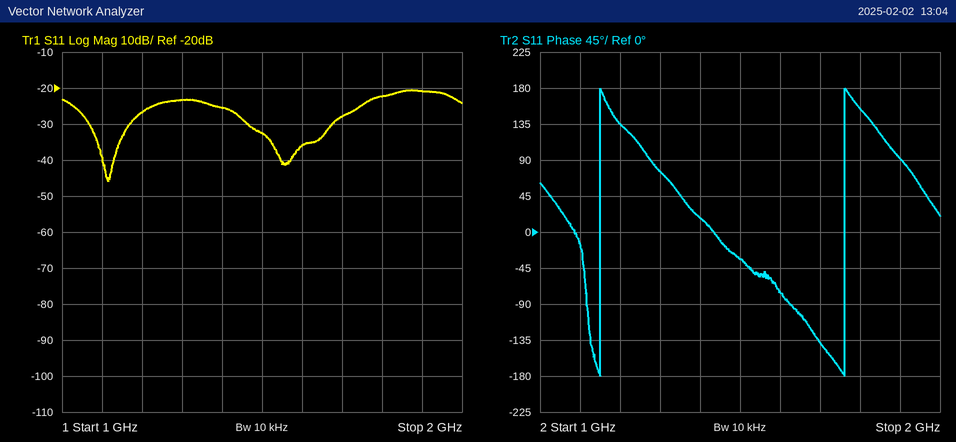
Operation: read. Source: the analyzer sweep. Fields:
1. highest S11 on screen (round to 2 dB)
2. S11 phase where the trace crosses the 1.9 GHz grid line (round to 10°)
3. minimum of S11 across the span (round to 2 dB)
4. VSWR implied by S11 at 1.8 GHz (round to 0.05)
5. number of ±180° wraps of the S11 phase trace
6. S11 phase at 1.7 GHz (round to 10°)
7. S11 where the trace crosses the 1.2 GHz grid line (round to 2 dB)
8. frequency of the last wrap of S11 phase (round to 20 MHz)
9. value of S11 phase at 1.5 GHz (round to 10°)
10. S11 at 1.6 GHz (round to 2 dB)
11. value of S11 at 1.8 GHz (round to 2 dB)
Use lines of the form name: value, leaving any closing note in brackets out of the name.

highest S11 on screen: -20 dB
S11 phase where the trace crosses the 1.9 GHz grid line: 90°
minimum of S11 across the span: -46 dB
VSWR implied by S11 at 1.8 GHz: 1.15
number of ±180° wraps of the S11 phase trace: 2
S11 phase at 1.7 GHz: -140°
S11 where the trace crosses the 1.2 GHz grid line: -26 dB
frequency of the last wrap of S11 phase: 1.76 GHz
value of S11 phase at 1.5 GHz: -30°
S11 at 1.6 GHz: -36 dB
value of S11 at 1.8 GHz: -22 dB
